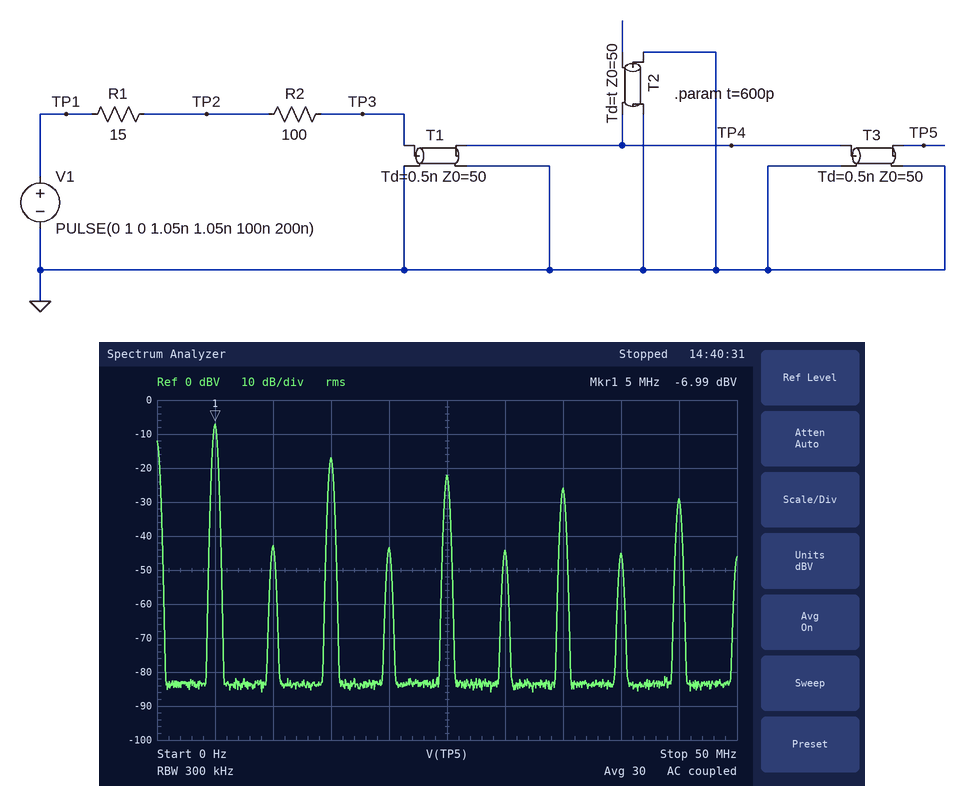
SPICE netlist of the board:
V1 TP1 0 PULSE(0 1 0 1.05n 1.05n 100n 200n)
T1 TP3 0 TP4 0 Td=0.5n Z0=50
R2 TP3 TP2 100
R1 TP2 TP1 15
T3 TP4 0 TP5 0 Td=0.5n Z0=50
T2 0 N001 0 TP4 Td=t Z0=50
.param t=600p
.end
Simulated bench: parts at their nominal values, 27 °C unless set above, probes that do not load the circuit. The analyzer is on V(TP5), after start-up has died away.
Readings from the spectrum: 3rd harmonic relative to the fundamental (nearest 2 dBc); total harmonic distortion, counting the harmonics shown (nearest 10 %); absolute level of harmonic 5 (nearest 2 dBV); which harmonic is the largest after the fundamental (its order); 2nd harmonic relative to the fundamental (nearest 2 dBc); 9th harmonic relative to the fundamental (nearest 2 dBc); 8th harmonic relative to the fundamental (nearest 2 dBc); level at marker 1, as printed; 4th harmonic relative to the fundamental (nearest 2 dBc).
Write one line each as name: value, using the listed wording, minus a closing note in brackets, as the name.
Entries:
3rd harmonic relative to the fundamental: -10 dBc
total harmonic distortion, counting the harmonics shown: 40 %
absolute level of harmonic 5: -22 dBV
which harmonic is the largest after the fundamental: 3
2nd harmonic relative to the fundamental: -36 dBc
9th harmonic relative to the fundamental: -22 dBc
8th harmonic relative to the fundamental: -38 dBc
level at marker 1, as printed: -6.99 dBV
4th harmonic relative to the fundamental: -36 dBc
